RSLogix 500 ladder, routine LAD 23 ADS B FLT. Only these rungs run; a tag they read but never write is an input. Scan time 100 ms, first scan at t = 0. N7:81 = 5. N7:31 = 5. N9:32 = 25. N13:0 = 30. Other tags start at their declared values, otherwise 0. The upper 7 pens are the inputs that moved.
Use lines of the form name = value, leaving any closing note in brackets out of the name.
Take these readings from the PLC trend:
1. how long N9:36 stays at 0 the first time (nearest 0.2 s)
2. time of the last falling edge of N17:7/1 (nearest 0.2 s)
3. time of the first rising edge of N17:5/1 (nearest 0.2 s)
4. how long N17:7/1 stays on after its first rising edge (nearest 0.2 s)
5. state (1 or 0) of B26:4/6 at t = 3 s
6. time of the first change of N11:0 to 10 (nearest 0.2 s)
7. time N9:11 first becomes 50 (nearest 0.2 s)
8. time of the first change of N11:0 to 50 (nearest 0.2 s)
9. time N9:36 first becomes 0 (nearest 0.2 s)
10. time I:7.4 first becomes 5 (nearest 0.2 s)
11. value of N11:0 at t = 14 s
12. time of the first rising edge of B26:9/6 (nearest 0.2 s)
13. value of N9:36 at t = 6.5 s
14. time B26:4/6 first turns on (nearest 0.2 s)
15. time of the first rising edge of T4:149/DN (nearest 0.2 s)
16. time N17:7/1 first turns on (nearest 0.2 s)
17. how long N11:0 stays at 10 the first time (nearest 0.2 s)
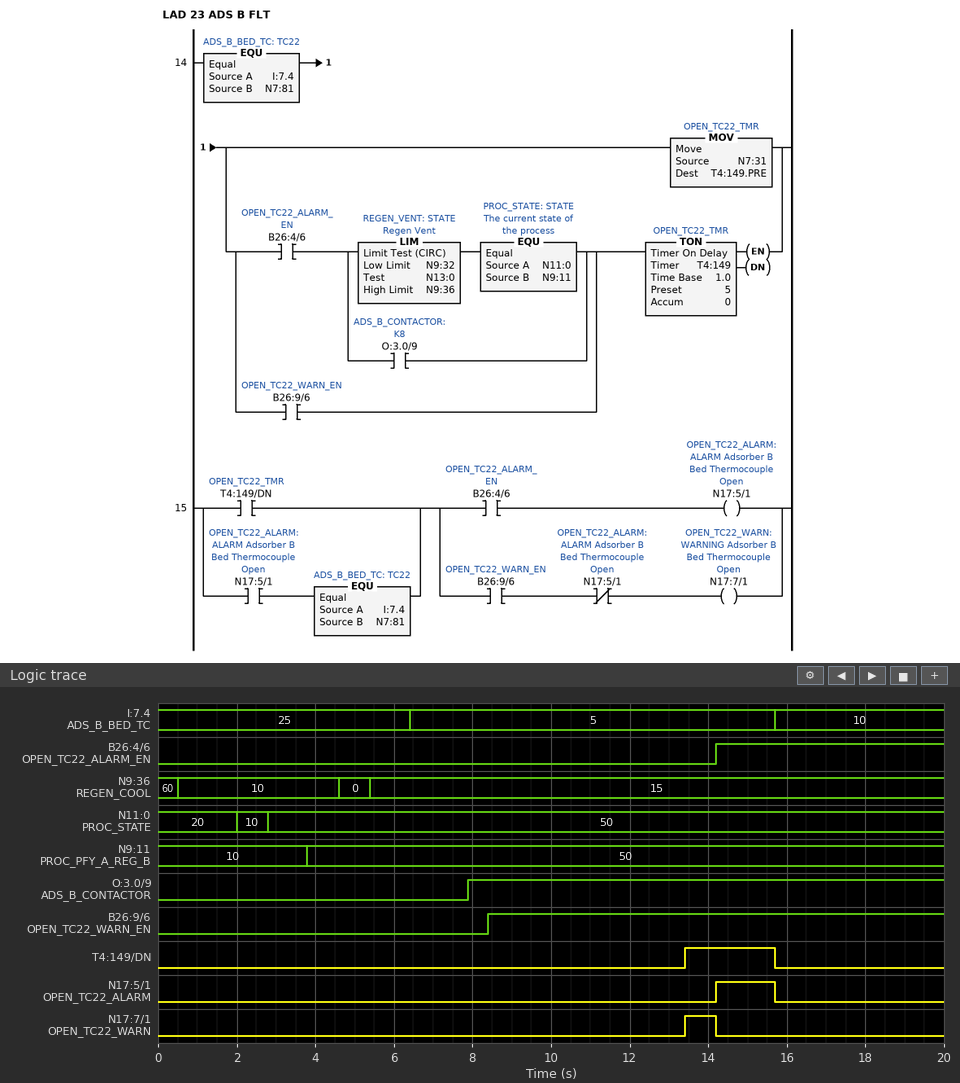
how long N9:36 stays at 0 the first time = 0.8 s
time of the last falling edge of N17:7/1 = 14.2 s
time of the first rising edge of N17:5/1 = 14.2 s
how long N17:7/1 stays on after its first rising edge = 0.8 s
state (1 or 0) of B26:4/6 at t = 3 s = 0
time of the first change of N11:0 to 10 = 2.0 s
time N9:11 first becomes 50 = 3.8 s
time of the first change of N11:0 to 50 = 2.8 s
time N9:36 first becomes 0 = 4.6 s
time I:7.4 first becomes 5 = 6.4 s
value of N11:0 at t = 14 s = 50
time of the first rising edge of B26:9/6 = 8.4 s
value of N9:36 at t = 6.5 s = 15
time B26:4/6 first turns on = 14.2 s
time of the first rising edge of T4:149/DN = 13.4 s
time N17:7/1 first turns on = 13.4 s
how long N11:0 stays at 10 the first time = 0.8 s
